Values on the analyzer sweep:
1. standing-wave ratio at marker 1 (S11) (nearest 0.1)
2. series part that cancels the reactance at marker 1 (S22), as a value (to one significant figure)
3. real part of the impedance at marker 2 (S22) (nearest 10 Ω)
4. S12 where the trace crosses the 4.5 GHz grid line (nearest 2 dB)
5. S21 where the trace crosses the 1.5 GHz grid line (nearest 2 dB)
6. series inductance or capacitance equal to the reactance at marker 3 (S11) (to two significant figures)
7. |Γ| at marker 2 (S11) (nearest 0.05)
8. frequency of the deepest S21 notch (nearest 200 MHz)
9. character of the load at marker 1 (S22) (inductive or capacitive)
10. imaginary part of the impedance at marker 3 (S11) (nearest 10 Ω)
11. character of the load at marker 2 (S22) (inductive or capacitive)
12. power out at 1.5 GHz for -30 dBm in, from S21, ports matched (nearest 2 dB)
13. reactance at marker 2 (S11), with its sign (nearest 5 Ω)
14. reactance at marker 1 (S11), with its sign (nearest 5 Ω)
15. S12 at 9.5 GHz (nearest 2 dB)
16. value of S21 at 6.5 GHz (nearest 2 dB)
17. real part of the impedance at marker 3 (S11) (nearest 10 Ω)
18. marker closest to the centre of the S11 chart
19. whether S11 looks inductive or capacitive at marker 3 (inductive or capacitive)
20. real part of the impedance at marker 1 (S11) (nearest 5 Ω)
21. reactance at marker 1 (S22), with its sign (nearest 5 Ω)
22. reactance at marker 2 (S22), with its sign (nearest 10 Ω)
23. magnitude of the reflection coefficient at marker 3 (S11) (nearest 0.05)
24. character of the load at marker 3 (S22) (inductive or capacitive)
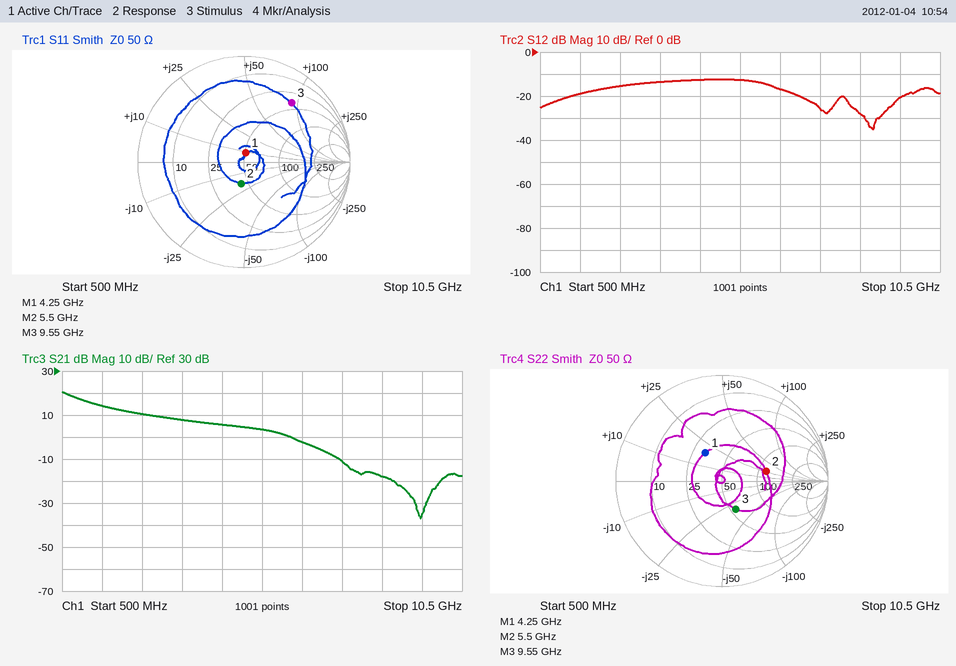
1.2
2 pF
120 Ω
-12 dB
14 dB
1.5 nH
0.20
9.4 GHz
inductive
+90 Ω
inductive
-16 dBm
-20 Ω
+10 Ω
-20 dB
-2 dB
40 Ω
marker 1
inductive
50 Ω
+20 Ω
+30 Ω
0.70
capacitive
